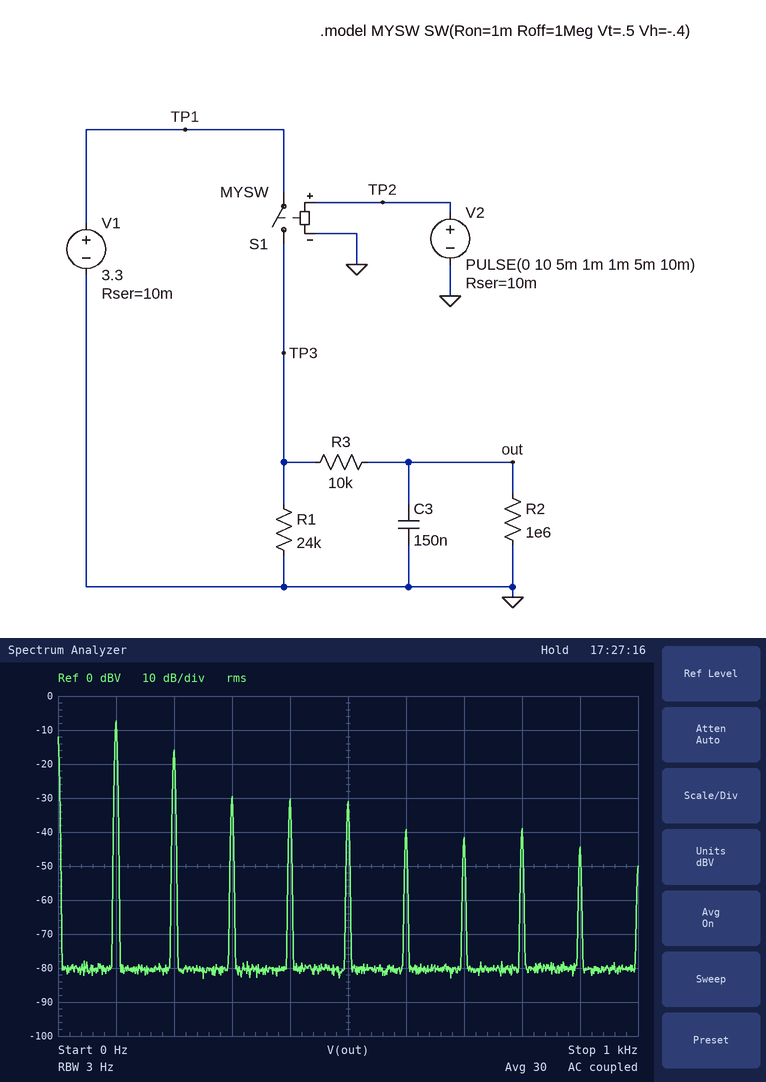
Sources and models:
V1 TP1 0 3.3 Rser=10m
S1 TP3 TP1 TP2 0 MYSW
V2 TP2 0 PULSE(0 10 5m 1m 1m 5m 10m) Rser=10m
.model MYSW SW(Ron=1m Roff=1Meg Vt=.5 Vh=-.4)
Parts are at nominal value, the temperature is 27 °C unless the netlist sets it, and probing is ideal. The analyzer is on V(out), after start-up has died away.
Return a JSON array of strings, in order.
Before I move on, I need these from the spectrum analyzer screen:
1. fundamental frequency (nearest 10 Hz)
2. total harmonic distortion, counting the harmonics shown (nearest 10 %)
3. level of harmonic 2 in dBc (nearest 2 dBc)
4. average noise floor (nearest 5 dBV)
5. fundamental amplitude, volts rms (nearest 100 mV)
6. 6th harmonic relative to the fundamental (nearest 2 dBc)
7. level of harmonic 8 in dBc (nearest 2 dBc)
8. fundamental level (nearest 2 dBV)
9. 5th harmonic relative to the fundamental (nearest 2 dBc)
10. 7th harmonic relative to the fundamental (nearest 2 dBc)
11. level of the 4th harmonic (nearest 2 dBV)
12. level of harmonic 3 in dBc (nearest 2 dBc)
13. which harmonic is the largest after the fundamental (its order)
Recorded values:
["100 Hz", "40 %", "-8 dBc", "-80 dBV", "400 mV", "-32 dBc", "-32 dBc", "-8 dBV", "-24 dBc", "-34 dBc", "-30 dBV", "-22 dBc", "2"]
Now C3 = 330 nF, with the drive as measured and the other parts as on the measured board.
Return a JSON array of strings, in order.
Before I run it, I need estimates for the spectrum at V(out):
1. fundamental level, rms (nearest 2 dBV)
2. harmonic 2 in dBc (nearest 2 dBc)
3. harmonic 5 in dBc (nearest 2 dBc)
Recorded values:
["-14 dBV", "-10 dBc", "-26 dBc"]
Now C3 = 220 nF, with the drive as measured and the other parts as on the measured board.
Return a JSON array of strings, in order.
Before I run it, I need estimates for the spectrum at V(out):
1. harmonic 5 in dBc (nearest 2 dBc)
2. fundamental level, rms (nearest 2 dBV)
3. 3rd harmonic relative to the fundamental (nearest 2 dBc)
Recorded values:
["-24 dBc", "-10 dBV", "-24 dBc"]
